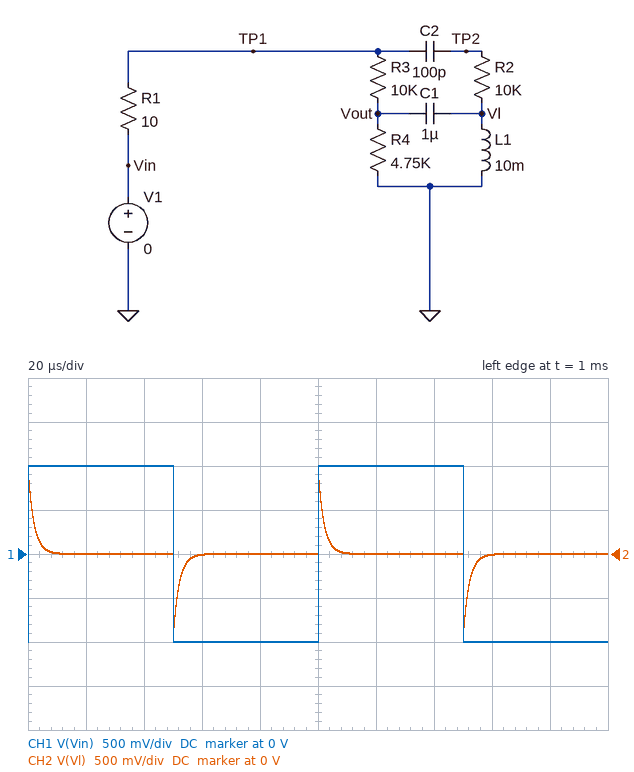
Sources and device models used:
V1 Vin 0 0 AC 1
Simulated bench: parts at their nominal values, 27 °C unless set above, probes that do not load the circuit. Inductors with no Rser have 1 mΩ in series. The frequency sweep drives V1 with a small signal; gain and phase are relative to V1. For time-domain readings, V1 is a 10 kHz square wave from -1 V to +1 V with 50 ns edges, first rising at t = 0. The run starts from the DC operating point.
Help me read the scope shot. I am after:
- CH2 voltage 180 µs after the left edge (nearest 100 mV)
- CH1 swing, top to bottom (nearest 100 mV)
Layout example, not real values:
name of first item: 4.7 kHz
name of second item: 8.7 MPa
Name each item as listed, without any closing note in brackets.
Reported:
CH2 voltage 180 µs after the left edge: 0 V
CH1 swing, top to bottom: 2.0 V
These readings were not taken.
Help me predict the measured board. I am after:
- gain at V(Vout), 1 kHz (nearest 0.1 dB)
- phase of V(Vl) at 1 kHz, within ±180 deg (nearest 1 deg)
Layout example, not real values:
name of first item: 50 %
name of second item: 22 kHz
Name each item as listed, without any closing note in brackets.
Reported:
gain at V(Vout), 1 kHz: -40.3 dB
phase of V(Vl) at 1 kHz, within ±180 deg: 92 deg
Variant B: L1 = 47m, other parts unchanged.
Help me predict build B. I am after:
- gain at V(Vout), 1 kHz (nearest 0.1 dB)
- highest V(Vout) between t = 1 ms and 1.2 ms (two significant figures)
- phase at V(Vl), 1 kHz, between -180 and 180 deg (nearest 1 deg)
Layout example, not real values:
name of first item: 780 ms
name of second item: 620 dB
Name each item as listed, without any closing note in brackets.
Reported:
gain at V(Vout), 1 kHz: -37.3 dB
highest V(Vout) between t = 1 ms and 1.2 ms: 720 mV
phase at V(Vl), 1 kHz, between -180 and 180 deg: 88 deg
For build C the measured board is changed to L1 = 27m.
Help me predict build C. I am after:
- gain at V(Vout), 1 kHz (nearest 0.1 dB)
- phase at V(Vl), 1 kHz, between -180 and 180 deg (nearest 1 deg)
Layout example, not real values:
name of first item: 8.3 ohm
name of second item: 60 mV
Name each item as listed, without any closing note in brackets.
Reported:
gain at V(Vout), 1 kHz: -59.5 dB
phase at V(Vl), 1 kHz, between -180 and 180 deg: 90 deg
